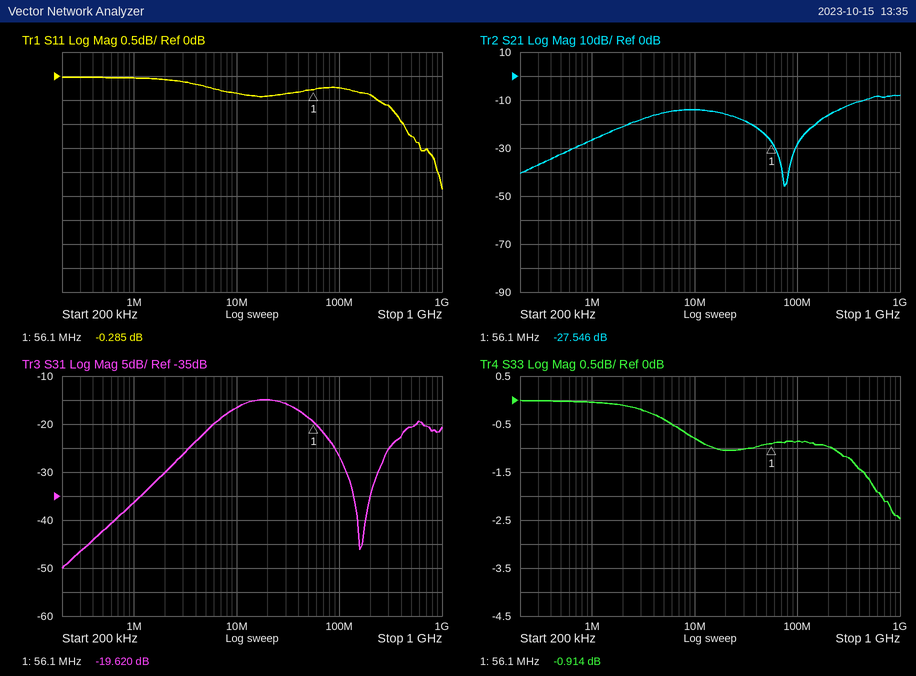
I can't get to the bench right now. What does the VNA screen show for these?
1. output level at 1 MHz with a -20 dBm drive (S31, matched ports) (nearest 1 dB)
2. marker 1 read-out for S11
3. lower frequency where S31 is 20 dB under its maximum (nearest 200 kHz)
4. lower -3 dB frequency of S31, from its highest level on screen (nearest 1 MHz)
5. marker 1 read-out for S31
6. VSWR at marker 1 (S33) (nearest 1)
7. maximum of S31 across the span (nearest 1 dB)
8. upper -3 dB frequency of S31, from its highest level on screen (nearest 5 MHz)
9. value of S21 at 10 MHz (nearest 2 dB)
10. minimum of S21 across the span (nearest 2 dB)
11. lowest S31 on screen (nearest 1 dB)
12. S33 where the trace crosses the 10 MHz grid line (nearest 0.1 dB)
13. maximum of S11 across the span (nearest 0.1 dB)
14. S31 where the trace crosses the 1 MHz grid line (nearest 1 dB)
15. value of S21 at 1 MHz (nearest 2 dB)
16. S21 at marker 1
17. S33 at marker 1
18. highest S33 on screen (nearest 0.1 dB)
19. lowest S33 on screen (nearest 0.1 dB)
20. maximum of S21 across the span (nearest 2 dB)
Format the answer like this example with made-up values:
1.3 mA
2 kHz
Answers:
-56 dBm
-0.285 dB
1.2 MHz
8 MHz
-19.620 dB
19
-15 dB
45 MHz
-14 dB
-46 dB
-50 dB
-0.8 dB
0.0 dB
-36 dB
-26 dB
-27.546 dB
-0.914 dB
0.0 dB
-2.5 dB
-8 dB
